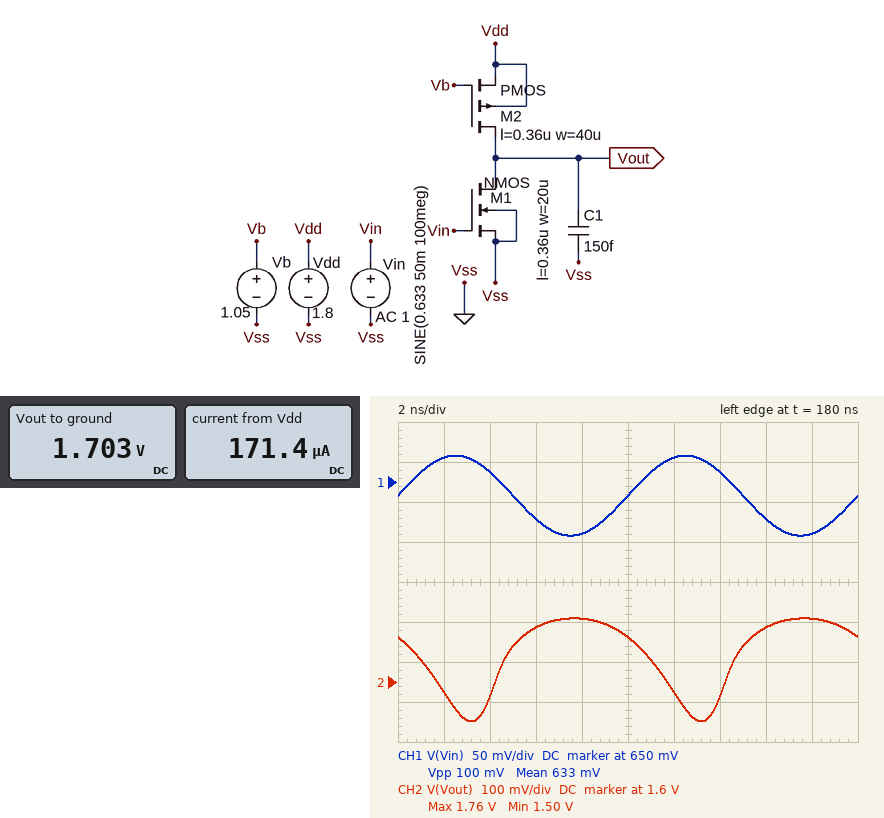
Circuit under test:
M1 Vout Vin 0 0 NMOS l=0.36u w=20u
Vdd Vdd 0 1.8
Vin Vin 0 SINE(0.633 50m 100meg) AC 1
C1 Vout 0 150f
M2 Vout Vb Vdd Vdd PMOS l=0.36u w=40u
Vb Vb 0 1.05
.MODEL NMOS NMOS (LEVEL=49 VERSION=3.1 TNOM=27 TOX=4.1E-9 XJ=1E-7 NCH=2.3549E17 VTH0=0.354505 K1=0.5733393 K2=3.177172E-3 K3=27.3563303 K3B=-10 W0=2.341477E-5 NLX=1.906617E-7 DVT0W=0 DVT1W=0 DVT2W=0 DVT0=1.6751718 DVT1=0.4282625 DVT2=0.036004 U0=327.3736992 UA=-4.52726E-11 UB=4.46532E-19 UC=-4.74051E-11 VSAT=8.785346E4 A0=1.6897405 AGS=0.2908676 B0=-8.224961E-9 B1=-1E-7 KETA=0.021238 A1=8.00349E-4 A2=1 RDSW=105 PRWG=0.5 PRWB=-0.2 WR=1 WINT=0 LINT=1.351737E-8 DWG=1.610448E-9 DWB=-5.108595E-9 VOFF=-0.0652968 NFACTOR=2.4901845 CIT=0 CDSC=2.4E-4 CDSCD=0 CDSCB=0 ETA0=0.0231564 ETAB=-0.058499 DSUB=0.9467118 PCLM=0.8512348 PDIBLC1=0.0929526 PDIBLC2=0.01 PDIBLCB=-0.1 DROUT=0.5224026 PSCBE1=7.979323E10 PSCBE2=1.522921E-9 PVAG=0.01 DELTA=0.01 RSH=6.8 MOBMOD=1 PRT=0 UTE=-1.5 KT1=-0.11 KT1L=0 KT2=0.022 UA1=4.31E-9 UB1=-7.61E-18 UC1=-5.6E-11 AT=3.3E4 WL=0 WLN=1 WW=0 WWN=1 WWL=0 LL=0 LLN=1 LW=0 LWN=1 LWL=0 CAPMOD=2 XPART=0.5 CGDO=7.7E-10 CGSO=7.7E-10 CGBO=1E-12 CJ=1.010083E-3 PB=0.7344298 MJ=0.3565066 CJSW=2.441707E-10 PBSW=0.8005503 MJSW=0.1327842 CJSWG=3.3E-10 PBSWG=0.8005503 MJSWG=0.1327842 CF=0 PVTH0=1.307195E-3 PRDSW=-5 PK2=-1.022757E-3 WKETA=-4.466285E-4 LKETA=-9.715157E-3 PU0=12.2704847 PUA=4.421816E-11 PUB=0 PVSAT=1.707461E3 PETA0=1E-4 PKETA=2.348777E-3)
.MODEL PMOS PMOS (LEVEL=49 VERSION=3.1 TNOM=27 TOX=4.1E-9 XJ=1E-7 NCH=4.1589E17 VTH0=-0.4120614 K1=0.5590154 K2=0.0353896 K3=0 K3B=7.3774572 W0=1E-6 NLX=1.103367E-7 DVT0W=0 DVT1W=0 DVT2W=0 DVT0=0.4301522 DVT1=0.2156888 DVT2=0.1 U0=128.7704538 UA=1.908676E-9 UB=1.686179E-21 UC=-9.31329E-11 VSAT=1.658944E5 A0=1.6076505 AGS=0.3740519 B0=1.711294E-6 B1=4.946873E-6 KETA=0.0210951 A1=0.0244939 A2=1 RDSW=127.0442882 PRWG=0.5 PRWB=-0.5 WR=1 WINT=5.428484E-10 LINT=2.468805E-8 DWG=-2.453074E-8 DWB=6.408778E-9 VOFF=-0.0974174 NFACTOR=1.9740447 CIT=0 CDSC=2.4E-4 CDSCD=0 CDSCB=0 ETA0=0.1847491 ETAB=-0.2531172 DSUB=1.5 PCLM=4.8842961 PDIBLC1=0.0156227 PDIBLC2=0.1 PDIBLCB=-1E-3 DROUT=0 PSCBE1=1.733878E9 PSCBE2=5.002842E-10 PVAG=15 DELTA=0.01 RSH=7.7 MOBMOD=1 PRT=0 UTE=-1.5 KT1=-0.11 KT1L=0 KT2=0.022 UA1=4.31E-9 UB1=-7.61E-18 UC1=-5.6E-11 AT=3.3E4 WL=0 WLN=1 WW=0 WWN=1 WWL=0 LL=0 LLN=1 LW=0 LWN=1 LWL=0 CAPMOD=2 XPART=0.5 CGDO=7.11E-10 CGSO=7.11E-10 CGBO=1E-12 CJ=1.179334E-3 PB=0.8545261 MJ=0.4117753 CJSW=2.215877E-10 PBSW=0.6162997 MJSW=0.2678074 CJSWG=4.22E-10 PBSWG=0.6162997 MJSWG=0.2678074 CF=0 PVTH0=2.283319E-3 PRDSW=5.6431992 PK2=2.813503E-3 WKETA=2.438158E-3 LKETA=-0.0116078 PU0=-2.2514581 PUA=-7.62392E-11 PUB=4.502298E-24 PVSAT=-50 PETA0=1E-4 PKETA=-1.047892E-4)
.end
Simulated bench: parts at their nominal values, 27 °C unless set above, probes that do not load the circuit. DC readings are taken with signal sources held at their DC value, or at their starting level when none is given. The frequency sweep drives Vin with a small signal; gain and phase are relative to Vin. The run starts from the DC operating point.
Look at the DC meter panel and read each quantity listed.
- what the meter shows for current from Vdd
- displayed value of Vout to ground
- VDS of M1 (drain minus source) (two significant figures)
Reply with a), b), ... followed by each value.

a) 171.4 µA
b) 1.703 V
c) 1.7 V
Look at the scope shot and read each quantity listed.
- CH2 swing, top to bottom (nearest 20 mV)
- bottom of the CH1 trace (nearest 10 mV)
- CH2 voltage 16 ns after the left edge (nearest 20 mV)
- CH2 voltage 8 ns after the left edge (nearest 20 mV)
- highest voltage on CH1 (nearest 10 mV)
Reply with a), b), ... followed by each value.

a) 260 mV
b) 580 mV
c) 1.74 V
d) 1.76 V
e) 680 mV
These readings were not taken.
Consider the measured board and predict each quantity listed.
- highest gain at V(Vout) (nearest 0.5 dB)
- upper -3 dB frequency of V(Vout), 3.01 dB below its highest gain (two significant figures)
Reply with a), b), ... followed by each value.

a) 4.5 dB
b) 900 MHz
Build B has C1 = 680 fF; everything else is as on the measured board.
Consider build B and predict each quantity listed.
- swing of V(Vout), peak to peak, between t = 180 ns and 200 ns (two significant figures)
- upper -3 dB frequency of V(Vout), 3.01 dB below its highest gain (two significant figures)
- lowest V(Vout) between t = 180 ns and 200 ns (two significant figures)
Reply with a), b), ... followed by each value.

a) 190 mV
b) 280 MHz
c) 1.6 V
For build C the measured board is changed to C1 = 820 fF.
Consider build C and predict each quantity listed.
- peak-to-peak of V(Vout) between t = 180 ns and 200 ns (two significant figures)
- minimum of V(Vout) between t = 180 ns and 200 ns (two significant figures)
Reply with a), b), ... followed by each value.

a) 180 mV
b) 1.6 V
